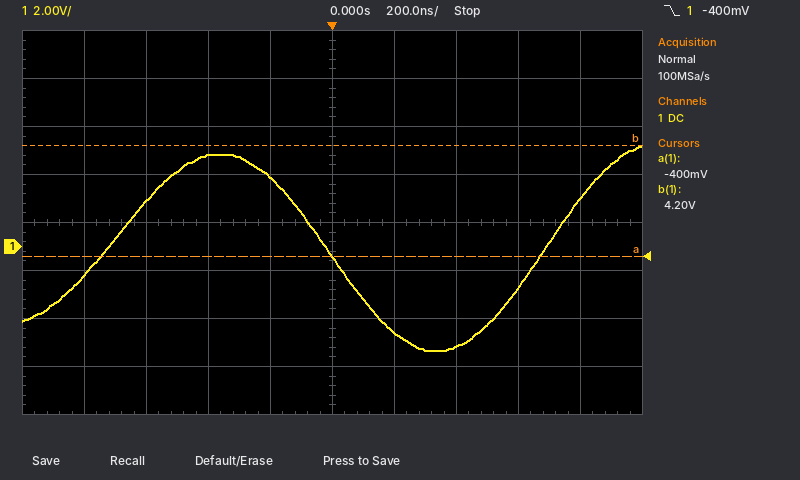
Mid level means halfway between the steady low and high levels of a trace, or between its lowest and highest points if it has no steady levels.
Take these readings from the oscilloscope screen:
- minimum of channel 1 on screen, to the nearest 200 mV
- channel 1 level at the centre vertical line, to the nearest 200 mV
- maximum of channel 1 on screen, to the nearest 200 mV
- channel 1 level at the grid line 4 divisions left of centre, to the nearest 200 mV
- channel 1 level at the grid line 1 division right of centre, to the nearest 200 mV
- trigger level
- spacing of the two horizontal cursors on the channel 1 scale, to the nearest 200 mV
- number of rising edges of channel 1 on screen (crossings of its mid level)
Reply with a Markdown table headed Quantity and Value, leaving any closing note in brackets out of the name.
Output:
| Quantity | Value |
|---|---|
| minimum of channel 1 on screen, to the nearest 200 mV | -4.4 V |
| channel 1 level at the centre vertical line, to the nearest 200 mV | -400 mV |
| maximum of channel 1 on screen, to the nearest 200 mV | 4.2 V |
| channel 1 level at the grid line 4 divisions left of centre, to the nearest 200 mV | -1.2 V |
| channel 1 level at the grid line 1 division right of centre, to the nearest 200 mV | -3.6 V |
| trigger level | -400 mV |
| spacing of the two horizontal cursors on the channel 1 scale, to the nearest 200 mV | 4.6 V |
| number of rising edges of channel 1 on screen | 2 |
